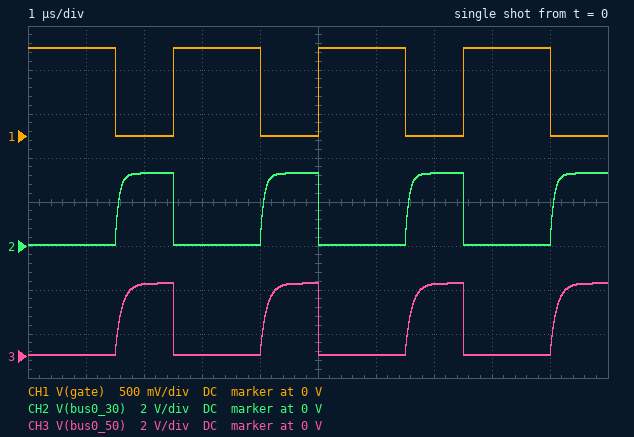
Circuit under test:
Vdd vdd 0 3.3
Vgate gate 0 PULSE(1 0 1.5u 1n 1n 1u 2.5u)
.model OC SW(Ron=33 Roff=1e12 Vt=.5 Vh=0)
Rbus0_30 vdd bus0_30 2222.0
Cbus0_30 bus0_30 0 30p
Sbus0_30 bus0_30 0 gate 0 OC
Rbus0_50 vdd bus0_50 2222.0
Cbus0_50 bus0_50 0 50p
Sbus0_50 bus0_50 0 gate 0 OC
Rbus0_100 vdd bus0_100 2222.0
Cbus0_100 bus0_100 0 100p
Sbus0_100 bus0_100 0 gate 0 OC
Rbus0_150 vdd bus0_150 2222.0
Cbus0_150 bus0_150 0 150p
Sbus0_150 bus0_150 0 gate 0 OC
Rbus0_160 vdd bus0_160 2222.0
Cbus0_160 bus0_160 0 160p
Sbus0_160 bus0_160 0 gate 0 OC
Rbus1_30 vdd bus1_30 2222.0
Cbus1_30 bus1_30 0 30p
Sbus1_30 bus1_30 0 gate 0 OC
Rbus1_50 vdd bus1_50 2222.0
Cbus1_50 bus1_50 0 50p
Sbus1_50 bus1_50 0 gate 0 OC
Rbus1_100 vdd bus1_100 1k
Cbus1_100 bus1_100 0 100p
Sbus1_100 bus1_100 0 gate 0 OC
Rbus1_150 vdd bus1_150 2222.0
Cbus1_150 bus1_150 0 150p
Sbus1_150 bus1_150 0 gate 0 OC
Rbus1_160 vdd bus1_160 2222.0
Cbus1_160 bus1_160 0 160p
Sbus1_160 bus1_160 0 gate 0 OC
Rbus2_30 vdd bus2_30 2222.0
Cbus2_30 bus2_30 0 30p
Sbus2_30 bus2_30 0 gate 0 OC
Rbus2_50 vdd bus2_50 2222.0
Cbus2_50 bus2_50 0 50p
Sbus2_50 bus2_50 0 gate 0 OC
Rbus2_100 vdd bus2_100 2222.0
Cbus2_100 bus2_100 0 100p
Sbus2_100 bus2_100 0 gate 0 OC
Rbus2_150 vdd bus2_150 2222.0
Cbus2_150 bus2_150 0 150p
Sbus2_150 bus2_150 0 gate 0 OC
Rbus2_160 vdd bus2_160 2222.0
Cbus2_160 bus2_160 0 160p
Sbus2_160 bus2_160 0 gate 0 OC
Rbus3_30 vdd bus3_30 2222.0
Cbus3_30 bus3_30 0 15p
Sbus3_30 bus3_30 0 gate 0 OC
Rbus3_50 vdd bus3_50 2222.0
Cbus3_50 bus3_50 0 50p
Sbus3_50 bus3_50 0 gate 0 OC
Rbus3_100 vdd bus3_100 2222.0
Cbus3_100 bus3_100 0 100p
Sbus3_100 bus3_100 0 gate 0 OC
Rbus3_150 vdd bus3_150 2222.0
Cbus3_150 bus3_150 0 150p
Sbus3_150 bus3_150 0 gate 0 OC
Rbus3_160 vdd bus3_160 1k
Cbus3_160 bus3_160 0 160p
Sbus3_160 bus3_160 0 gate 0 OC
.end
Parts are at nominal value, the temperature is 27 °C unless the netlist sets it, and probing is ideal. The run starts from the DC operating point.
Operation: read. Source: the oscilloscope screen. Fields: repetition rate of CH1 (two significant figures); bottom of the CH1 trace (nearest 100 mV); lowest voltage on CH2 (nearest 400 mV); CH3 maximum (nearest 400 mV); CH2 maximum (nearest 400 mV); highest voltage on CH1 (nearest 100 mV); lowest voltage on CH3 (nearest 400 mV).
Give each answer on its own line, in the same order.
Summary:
400 kHz
0 V
0 V
3.2 V
3.2 V
1.0 V
0 V
